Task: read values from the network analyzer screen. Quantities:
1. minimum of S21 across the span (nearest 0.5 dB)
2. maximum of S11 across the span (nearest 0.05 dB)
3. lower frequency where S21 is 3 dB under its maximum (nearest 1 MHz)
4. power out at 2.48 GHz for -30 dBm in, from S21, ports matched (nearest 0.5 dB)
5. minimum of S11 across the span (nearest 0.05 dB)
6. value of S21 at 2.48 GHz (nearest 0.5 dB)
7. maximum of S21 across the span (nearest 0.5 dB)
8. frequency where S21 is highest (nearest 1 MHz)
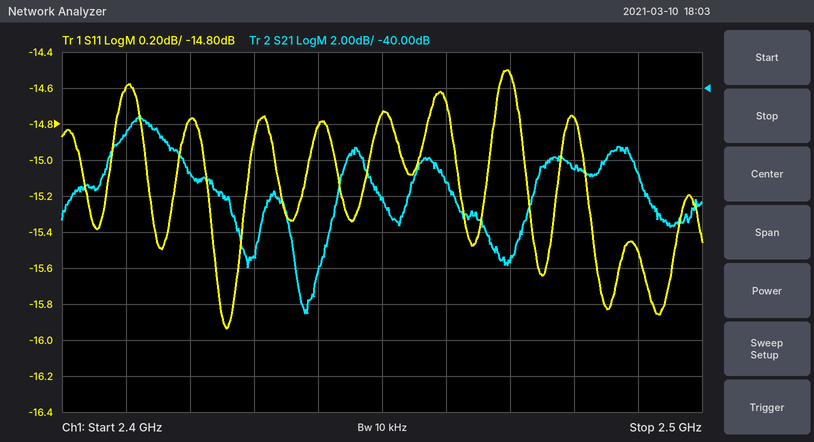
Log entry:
-52.5 dB
-14.50 dB
2.407 GHz
-74.5 dBm
-15.95 dB
-44.5 dB
-41.5 dB
2.412 GHz
